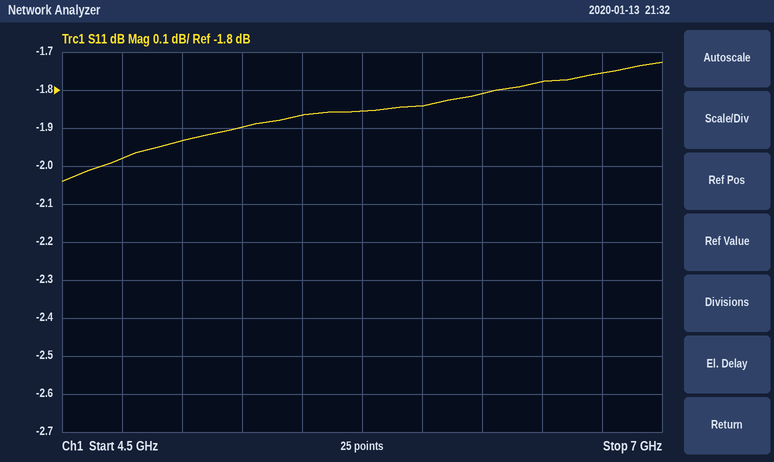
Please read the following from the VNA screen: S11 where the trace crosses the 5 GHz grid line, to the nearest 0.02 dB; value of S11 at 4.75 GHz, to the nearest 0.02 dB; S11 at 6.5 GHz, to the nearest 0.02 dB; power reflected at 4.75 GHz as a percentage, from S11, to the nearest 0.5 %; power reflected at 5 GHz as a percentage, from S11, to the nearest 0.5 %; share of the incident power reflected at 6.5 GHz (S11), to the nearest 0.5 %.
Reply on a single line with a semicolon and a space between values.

-1.94 dB; -1.98 dB; -1.78 dB; 63.5 %; 64.0 %; 66.5 %
